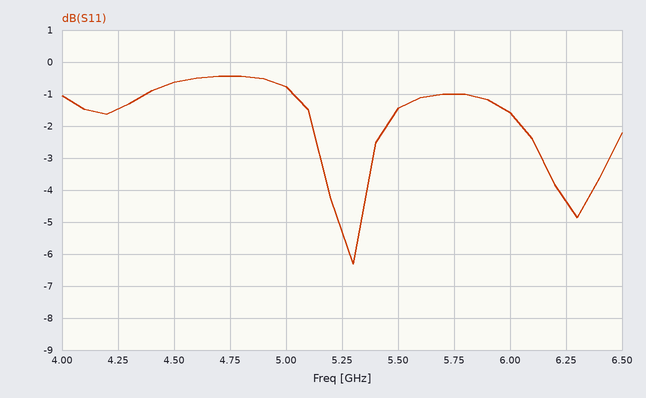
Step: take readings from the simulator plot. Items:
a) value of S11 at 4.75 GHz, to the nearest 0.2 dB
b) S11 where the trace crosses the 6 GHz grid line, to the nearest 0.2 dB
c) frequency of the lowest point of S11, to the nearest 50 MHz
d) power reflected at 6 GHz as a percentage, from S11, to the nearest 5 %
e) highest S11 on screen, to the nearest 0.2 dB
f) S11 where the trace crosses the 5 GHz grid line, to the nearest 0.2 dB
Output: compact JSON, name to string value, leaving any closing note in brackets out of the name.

{"value of S11 at 4.75 GHz, to the nearest 0.2 dB": "-0.4 dB", "S11 where the trace crosses the 6 GHz grid line, to the nearest 0.2 dB": "-1.6 dB", "frequency of the lowest point of S11, to the nearest 50 MHz": "5.30 GHz", "power reflected at 6 GHz as a percentage, from S11, to the nearest 5 %": "70 %", "highest S11 on screen, to the nearest 0.2 dB": "-0.4 dB", "S11 where the trace crosses the 5 GHz grid line, to the nearest 0.2 dB": "-0.8 dB"}
